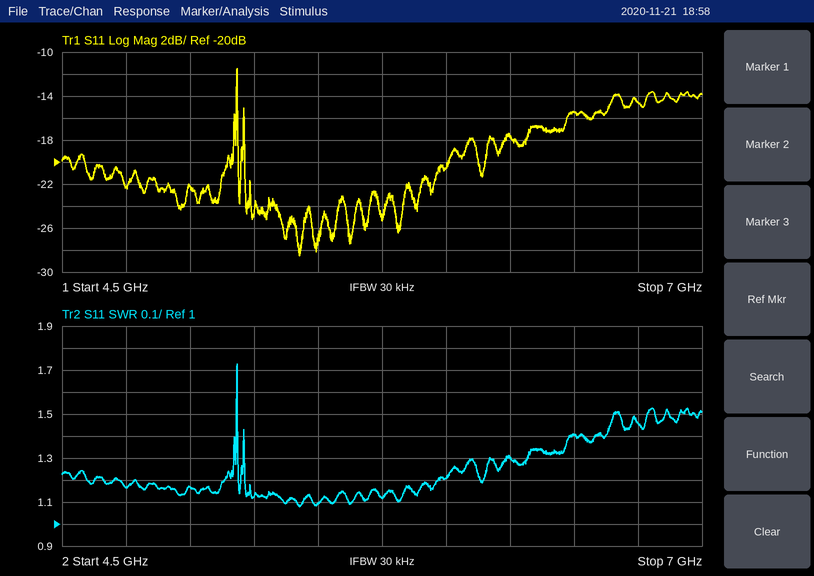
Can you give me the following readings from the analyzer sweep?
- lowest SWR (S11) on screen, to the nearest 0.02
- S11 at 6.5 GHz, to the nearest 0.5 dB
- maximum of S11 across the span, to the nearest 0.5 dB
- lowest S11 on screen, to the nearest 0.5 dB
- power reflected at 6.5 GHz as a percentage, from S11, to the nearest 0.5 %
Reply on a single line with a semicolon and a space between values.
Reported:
1.08; -15.5 dB; -11.5 dB; -28.5 dB; 3.0 %
